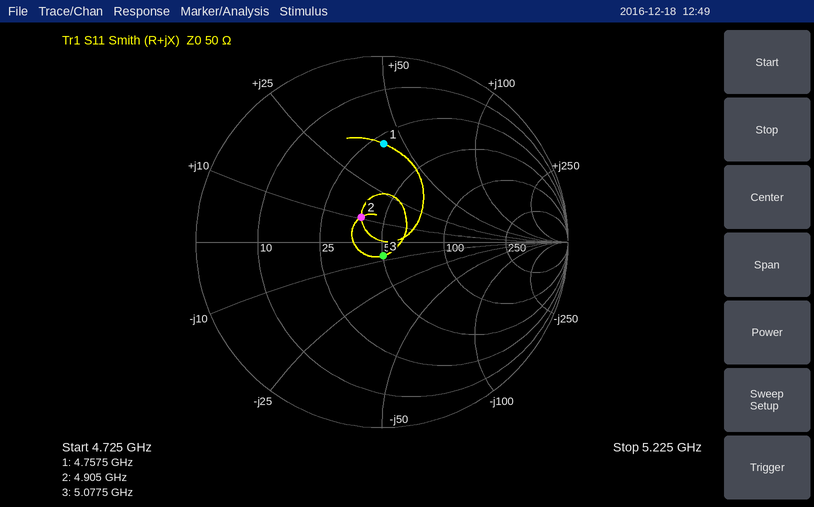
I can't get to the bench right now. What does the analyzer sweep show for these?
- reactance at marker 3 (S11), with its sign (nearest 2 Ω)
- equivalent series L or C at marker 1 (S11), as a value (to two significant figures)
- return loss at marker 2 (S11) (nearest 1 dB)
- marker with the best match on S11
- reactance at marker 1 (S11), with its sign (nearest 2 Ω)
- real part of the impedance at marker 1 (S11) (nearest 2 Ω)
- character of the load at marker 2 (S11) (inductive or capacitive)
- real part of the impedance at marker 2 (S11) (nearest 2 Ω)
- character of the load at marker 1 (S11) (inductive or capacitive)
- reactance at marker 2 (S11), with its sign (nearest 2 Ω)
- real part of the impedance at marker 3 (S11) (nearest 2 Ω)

-8 Ω
1.4 nH
15 dB
marker 3
+42 Ω
28 Ω
inductive
38 Ω
inductive
+10 Ω
50 Ω
